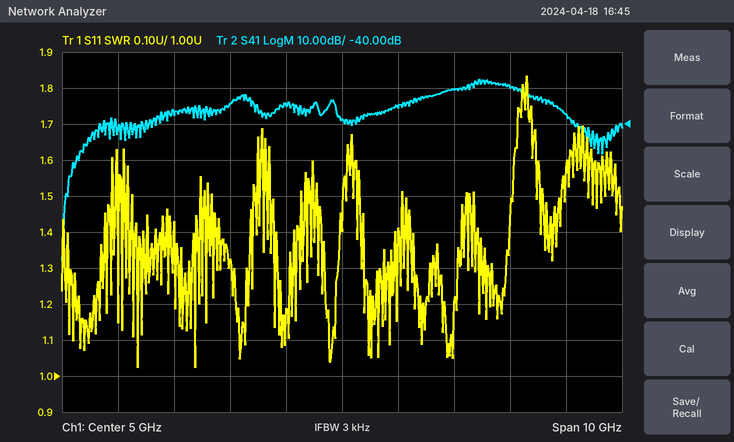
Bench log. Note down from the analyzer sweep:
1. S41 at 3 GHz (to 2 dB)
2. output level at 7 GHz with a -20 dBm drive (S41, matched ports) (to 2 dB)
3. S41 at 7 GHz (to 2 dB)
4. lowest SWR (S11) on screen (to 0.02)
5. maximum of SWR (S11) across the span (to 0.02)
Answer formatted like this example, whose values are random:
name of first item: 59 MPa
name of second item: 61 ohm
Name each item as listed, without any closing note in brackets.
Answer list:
S41 at 3 GHz: -34 dB
output level at 7 GHz with a -20 dBm drive (S41, matched ports): -50 dBm
S41 at 7 GHz: -30 dB
lowest SWR (S11) on screen: 1.02
maximum of SWR (S11) across the span: 1.84
